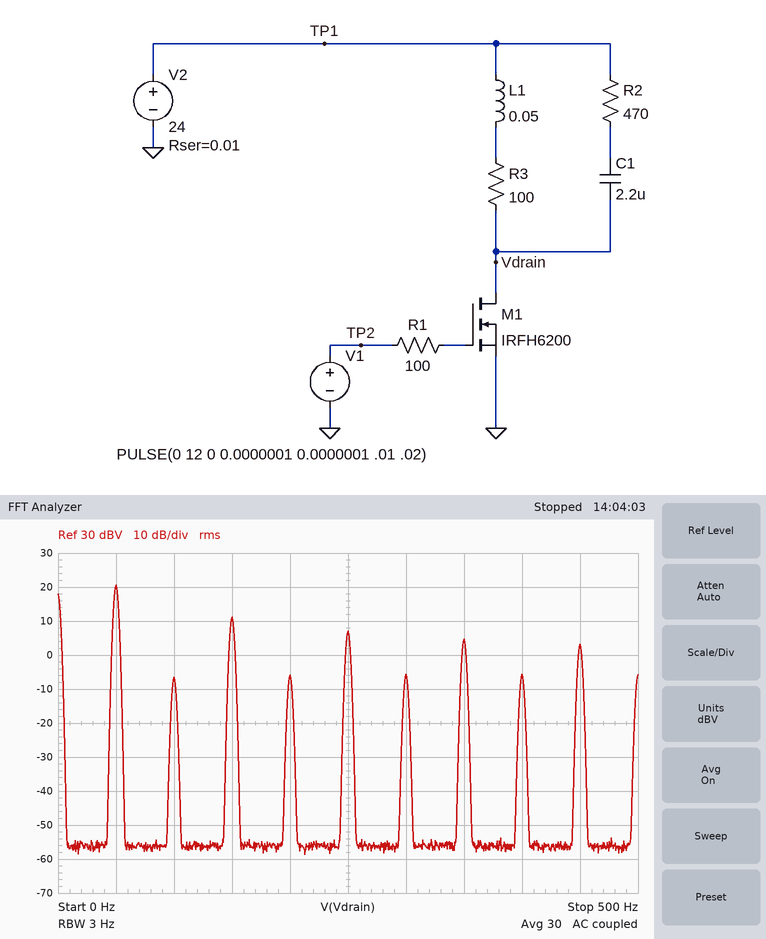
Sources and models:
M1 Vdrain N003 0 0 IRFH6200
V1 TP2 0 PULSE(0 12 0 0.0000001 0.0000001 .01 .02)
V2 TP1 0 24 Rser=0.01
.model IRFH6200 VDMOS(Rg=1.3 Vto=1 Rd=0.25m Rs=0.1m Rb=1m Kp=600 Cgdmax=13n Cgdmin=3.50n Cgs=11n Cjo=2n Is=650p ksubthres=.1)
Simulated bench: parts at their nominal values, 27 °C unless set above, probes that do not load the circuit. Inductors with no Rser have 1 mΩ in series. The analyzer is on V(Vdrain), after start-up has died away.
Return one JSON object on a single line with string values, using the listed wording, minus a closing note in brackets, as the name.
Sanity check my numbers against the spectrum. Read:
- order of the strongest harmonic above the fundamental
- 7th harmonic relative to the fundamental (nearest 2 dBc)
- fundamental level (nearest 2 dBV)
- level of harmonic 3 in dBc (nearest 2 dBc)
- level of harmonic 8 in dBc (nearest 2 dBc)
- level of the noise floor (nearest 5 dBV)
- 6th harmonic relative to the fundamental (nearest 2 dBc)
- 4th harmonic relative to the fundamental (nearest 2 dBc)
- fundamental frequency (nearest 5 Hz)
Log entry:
{"order of the strongest harmonic above the fundamental": "3", "7th harmonic relative to the fundamental": "-16 dBc", "fundamental level": "20 dBV", "level of harmonic 3 in dBc": "-10 dBc", "level of harmonic 8 in dBc": "-26 dBc", "level of the noise floor": "-55 dBV", "6th harmonic relative to the fundamental": "-26 dBc", "4th harmonic relative to the fundamental": "-26 dBc", "fundamental frequency": "50 Hz"}
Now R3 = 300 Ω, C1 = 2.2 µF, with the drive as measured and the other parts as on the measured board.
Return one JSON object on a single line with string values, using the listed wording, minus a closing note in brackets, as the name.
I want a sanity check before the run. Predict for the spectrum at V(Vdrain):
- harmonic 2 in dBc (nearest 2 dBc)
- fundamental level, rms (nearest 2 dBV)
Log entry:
{"harmonic 2 in dBc": "-24 dBc", "fundamental level, rms": "20 dBV"}
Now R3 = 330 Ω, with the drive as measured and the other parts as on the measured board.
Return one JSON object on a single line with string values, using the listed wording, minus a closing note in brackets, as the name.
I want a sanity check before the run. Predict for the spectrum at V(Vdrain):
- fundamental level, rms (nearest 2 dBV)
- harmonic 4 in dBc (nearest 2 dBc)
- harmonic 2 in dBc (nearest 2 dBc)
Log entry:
{"fundamental level, rms": "20 dBV", "harmonic 4 in dBc": "-28 dBc", "harmonic 2 in dBc": "-24 dBc"}
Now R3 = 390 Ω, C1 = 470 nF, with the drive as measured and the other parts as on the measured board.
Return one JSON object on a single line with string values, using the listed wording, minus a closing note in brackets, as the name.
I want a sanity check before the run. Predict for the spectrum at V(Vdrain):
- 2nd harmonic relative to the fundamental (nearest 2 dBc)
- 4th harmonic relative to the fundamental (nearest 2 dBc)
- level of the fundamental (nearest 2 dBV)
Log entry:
{"2nd harmonic relative to the fundamental": "-40 dBc", "4th harmonic relative to the fundamental": "-40 dBc", "level of the fundamental": "20 dBV"}
